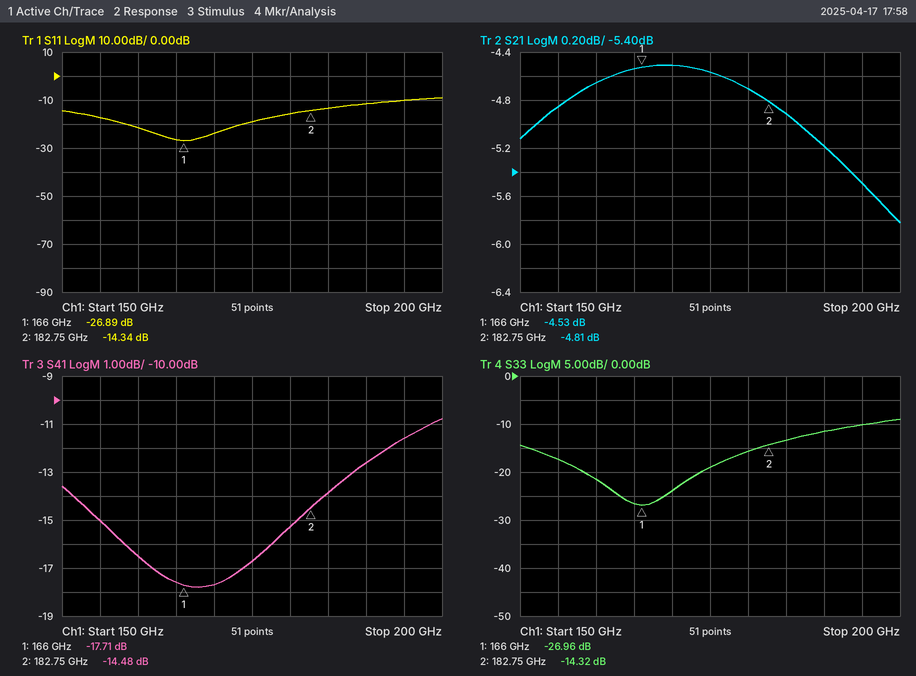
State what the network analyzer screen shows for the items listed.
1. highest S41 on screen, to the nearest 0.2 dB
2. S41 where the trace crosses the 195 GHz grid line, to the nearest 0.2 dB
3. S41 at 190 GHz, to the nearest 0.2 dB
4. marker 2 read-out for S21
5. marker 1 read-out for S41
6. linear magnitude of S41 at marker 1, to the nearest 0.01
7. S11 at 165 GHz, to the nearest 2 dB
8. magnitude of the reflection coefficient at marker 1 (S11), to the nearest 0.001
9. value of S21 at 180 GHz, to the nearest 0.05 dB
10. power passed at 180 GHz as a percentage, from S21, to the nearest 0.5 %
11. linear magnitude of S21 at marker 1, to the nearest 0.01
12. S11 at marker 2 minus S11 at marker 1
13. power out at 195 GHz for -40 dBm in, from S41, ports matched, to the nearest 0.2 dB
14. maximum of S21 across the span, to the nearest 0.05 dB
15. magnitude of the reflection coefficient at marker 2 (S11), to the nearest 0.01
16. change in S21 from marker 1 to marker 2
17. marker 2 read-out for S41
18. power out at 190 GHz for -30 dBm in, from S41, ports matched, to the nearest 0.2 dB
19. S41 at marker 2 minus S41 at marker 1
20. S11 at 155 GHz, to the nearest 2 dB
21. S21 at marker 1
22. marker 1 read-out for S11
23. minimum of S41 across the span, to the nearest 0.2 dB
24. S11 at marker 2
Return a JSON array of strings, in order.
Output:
["-10.8 dB", "-11.6 dB", "-12.6 dB", "-4.81 dB", "-17.71 dB", "0.13", "-26 dB", "0.045", "-4.70 dB", "34.0 %", "0.59", "12.55 dB", "-51.6 dBm", "-4.50 dB", "0.19", "-0.28 dB", "-14.48 dB", "-42.6 dBm", "3.23 dB", "-18 dB", "-4.53 dB", "-26.89 dB", "-17.8 dB", "-14.34 dB"]
